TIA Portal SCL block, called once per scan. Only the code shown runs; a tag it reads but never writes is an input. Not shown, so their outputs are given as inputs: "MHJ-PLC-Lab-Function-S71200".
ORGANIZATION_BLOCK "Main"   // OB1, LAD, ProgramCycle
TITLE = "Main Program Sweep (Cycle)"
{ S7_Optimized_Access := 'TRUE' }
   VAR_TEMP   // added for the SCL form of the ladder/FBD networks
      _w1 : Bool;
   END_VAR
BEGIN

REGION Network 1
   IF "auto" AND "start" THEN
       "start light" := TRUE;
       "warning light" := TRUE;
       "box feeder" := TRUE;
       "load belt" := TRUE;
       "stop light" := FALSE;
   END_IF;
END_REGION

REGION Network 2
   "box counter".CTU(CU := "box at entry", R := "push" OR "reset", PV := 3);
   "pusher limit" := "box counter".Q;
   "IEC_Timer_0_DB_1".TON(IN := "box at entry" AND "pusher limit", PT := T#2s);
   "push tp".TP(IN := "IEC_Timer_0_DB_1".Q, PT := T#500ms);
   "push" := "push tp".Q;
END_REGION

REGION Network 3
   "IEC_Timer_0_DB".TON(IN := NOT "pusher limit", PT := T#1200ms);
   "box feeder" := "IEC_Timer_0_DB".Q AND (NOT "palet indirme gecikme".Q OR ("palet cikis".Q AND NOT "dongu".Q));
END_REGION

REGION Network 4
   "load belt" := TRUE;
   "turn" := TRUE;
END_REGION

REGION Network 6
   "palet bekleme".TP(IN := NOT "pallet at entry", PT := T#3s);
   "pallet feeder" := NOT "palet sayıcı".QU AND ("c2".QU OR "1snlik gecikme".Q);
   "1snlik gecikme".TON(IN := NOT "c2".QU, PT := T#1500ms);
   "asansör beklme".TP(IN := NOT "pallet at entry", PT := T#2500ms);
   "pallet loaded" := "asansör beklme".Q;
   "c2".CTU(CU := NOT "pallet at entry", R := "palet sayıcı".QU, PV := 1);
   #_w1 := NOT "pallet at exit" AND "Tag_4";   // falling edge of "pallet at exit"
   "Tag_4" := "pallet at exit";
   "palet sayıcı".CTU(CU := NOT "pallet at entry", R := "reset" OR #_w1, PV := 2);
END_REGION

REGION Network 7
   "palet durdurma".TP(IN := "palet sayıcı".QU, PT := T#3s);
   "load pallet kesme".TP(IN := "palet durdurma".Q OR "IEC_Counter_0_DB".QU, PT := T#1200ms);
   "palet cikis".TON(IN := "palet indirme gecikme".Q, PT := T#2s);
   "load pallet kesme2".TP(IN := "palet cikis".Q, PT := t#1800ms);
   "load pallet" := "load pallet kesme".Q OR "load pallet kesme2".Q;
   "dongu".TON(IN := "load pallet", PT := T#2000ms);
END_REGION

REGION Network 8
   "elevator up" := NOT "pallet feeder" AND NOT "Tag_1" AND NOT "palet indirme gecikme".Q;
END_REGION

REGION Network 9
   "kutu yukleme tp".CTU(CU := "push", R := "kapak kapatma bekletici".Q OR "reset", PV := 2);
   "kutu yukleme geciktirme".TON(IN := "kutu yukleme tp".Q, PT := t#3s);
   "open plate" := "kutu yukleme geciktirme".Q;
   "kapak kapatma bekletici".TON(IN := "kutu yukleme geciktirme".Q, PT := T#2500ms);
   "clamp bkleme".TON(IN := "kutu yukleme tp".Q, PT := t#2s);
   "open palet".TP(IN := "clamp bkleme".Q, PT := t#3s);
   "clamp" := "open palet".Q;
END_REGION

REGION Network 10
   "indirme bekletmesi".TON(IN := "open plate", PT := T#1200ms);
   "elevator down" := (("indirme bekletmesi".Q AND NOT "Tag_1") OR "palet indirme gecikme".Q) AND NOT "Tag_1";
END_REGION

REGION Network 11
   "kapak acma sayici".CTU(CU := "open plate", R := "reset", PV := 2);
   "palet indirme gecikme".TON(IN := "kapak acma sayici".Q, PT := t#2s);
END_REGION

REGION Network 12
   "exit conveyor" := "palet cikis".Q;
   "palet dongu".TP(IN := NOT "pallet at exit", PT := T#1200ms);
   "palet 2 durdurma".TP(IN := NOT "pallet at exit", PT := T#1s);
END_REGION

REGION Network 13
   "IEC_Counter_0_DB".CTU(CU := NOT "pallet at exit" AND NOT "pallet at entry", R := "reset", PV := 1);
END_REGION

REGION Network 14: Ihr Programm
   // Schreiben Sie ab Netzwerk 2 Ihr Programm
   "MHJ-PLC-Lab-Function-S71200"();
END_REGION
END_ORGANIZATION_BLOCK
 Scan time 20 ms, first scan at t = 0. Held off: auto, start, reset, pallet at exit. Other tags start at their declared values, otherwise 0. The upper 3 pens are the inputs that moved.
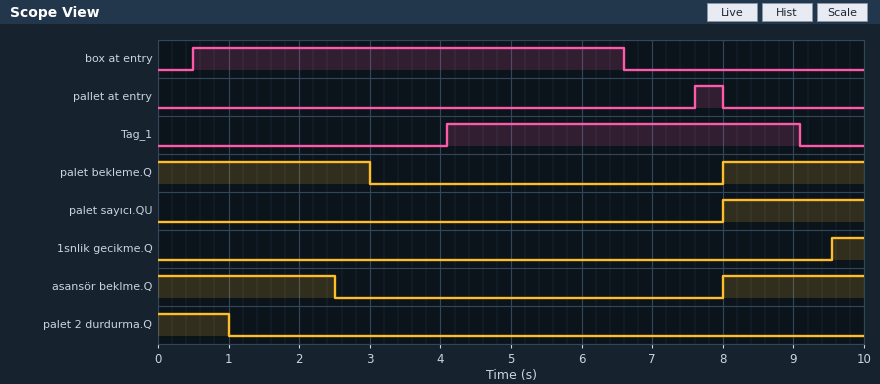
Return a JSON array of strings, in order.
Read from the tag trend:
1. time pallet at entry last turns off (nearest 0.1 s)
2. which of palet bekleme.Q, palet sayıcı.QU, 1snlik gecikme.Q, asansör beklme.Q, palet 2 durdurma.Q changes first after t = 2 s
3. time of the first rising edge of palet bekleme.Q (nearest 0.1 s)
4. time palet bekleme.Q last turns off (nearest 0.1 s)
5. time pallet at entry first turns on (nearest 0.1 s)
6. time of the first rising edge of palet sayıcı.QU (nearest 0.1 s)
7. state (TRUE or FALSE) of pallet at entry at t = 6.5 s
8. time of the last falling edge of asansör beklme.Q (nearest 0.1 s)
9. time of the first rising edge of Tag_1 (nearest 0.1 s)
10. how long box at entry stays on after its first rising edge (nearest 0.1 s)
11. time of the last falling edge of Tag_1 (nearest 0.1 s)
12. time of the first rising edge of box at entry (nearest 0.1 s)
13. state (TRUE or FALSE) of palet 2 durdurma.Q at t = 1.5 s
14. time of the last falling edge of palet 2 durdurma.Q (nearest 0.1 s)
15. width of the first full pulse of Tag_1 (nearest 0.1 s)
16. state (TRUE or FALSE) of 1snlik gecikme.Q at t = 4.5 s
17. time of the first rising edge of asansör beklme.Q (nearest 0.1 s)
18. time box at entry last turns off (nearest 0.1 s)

["8.0 s", "asansör beklme.Q", "8.0 s", "3.0 s", "7.6 s", "8.0 s", "FALSE", "2.5 s", "4.1 s", "6.1 s", "9.1 s", "0.5 s", "FALSE", "1.0 s", "5.0 s", "FALSE", "8.0 s", "6.6 s"]
